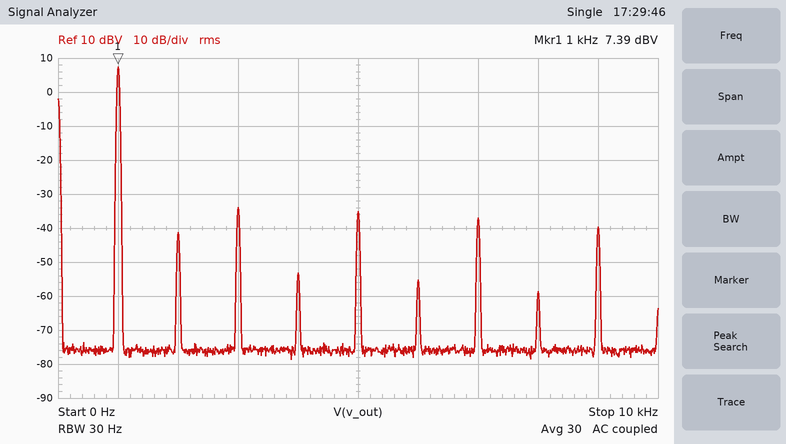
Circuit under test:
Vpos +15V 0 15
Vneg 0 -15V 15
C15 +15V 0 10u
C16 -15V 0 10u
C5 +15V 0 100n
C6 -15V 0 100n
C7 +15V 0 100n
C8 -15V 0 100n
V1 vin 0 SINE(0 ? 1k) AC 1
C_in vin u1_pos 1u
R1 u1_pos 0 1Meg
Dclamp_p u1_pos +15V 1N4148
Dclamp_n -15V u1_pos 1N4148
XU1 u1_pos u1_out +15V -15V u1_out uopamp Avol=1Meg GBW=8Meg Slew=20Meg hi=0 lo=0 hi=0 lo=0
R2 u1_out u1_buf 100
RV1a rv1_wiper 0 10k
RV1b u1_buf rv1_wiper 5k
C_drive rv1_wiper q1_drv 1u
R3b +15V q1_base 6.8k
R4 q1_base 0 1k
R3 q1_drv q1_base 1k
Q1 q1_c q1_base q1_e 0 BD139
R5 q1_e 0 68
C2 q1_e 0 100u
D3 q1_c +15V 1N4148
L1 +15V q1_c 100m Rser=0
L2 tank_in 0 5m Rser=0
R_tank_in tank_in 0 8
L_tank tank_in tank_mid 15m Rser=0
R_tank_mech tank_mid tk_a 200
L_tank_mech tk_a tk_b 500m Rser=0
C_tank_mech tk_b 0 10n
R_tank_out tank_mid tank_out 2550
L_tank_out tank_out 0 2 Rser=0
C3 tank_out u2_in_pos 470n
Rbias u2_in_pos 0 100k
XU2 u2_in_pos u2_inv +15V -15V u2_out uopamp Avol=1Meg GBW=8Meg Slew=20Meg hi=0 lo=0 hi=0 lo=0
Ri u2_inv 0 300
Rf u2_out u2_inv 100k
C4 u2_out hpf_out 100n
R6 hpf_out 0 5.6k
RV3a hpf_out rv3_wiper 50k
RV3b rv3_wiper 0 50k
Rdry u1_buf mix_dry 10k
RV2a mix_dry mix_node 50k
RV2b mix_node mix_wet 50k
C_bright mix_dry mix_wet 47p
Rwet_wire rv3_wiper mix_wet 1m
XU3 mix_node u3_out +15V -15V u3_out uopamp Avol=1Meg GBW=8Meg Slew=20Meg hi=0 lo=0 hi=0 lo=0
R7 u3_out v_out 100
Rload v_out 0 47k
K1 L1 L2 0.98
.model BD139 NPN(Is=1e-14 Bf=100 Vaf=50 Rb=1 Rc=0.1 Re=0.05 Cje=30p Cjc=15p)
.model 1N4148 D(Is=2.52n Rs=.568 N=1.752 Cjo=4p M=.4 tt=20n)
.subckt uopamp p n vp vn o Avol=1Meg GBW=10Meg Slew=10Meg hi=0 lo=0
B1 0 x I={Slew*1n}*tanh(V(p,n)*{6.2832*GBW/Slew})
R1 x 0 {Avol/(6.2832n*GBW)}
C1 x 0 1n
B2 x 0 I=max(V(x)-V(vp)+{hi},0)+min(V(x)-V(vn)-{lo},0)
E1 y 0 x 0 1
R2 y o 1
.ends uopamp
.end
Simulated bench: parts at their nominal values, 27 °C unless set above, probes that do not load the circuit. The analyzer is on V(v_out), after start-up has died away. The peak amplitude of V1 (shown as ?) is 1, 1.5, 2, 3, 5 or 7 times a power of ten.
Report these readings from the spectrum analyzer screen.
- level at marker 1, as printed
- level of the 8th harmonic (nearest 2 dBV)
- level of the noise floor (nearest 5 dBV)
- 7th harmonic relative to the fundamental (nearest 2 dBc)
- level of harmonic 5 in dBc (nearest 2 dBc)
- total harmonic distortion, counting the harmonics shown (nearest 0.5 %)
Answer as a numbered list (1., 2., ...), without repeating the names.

1. 7.39 dBV
2. -58 dBV
3. -75 dBV
4. -44 dBc
5. -42 dBc
6. 1.5 %
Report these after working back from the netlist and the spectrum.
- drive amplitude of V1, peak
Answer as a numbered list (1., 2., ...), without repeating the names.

1. 100 mV
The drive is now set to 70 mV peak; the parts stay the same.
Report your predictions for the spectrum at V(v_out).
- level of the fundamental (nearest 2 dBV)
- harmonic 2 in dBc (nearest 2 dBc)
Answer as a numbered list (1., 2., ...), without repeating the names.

1. 4 dBV
2. -50 dBc
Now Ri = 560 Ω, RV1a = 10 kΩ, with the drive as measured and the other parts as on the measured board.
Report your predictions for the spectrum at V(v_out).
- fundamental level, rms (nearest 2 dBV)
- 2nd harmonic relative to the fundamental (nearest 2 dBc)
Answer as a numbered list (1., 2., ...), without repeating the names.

1. 2 dBV
2. -48 dBc
